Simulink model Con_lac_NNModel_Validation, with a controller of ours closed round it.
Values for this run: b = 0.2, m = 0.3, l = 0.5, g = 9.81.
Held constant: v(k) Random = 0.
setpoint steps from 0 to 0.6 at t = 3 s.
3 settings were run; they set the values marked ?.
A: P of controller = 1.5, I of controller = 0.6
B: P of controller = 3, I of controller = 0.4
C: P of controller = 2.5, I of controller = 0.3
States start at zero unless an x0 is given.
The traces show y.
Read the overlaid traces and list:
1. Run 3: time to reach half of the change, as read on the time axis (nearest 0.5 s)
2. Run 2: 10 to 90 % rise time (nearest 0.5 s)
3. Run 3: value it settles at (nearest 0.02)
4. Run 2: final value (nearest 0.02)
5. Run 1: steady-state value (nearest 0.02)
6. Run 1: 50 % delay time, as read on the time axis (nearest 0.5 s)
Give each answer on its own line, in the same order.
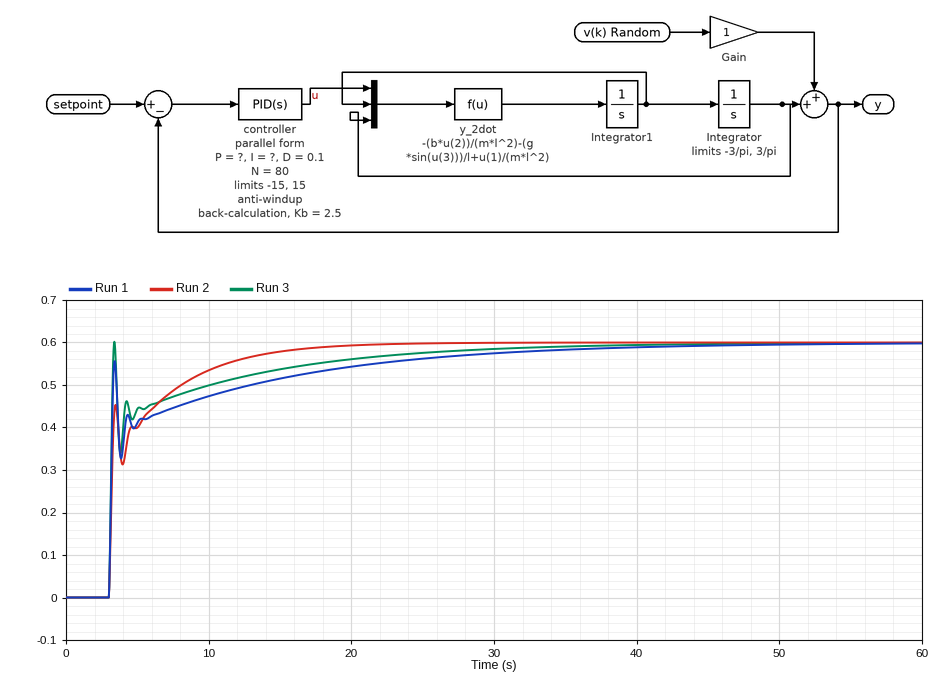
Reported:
3.0 s
7.5 s
0.60
0.60
0.60
3.0 s
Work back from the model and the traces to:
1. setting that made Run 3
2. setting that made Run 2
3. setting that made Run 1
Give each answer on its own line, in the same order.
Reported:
B
A
C
